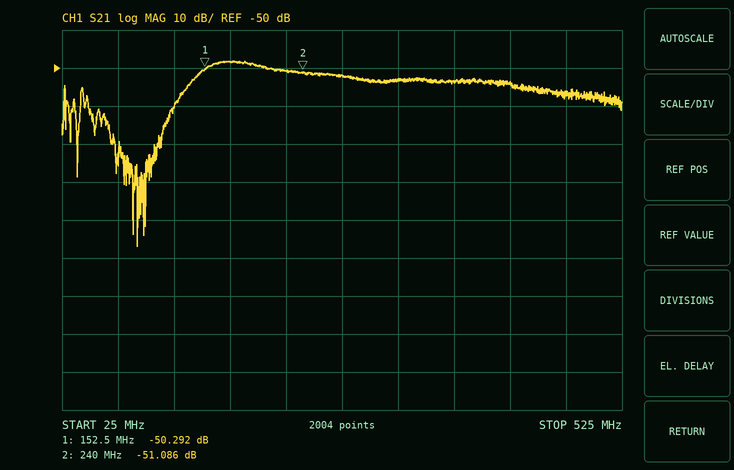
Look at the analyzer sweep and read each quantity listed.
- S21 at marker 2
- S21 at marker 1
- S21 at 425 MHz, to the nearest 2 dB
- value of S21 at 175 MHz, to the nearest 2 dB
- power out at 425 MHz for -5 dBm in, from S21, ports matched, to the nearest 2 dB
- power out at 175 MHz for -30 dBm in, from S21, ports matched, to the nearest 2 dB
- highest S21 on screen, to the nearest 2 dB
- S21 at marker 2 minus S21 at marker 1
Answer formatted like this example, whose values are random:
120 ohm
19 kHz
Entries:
-51.086 dB
-50.292 dB
-54 dB
-48 dB
-58 dBm
-78 dBm
-48 dB
-0.794 dB
